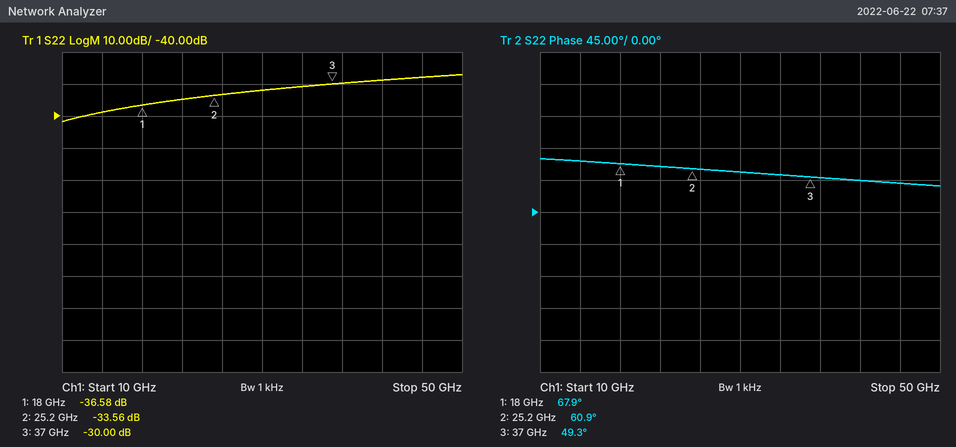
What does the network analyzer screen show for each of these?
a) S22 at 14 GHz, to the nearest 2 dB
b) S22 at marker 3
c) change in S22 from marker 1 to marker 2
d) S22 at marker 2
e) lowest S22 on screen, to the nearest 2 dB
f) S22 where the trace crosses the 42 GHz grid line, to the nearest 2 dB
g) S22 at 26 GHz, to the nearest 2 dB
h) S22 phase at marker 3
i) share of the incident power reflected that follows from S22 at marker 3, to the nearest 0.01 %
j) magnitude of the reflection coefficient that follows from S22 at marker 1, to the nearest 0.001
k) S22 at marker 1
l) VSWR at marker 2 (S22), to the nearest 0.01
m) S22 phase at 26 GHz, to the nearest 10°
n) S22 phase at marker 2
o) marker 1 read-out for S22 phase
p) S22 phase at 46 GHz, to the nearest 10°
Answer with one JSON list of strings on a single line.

["-38 dB", "-30.00 dB", "3.02 dB", "-33.56 dB", "-42 dB", "-28 dB", "-34 dB", "49.3°", "0.10 %", "0.015", "-36.58 dB", "1.04", "60°", "60.9°", "67.9°", "40°"]
